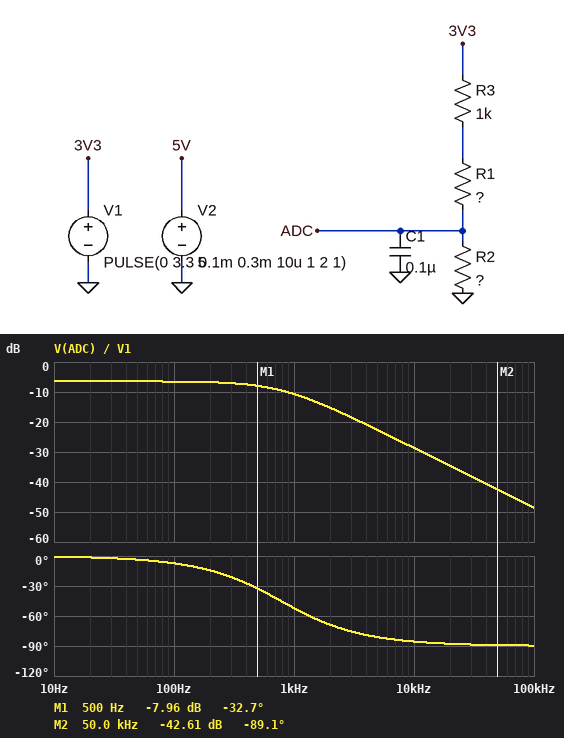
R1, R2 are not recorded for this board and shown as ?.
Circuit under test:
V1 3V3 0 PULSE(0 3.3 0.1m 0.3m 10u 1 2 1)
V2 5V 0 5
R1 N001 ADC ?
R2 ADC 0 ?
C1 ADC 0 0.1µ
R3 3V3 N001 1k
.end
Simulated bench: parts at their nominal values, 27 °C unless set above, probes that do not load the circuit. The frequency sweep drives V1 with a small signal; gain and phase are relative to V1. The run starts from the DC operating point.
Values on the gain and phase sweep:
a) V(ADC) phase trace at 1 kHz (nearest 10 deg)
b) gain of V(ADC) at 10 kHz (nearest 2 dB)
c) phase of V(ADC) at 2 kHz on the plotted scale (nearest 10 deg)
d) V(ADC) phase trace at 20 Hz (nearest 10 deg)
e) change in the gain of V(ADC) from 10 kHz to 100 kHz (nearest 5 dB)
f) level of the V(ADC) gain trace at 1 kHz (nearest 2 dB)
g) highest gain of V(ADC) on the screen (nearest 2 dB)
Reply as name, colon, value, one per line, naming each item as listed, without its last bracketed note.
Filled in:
V(ADC) phase trace at 1 kHz: -50 deg
gain of V(ADC) at 10 kHz: -28 dB
phase of V(ADC) at 2 kHz on the plotted scale: -70 deg
V(ADC) phase trace at 20 Hz: 0 deg
change in the gain of V(ADC) from 10 kHz to 100 kHz: -20 dB
level of the V(ADC) gain trace at 1 kHz: -10 dB
highest gain of V(ADC) on the screen: -6 dB
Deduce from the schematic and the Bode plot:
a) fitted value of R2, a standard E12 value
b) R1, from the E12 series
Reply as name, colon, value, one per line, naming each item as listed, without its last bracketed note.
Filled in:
fitted value of R2, a standard E12 value: 3.9 kΩ
R1, from the E12 series: 3.3 kΩ
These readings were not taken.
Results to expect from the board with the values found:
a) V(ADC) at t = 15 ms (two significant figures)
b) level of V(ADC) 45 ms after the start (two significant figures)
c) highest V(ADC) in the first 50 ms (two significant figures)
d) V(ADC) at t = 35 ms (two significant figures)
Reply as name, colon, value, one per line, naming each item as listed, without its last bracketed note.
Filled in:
V(ADC) at t = 15 ms: 1.6 V
level of V(ADC) 45 ms after the start: 1.6 V
highest V(ADC) in the first 50 ms: 1.6 V
V(ADC) at t = 35 ms: 1.6 V
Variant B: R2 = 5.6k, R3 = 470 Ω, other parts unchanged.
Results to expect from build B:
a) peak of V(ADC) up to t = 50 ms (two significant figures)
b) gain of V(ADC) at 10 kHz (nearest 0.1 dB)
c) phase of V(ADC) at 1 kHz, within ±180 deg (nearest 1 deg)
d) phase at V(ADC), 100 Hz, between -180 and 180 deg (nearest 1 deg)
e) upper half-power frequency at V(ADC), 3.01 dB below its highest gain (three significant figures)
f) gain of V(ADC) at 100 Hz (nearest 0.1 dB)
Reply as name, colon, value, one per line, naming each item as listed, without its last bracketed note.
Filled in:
peak of V(ADC) up to t = 50 ms: 2.0 V
gain of V(ADC) at 10 kHz: -27.5 dB
phase of V(ADC) at 1 kHz, within ±180 deg: -55 deg
phase at V(ADC), 100 Hz, between -180 and 180 deg: -8 deg
upper half-power frequency at V(ADC), 3.01 dB below its highest gain: 706 Hz
gain of V(ADC) at 100 Hz: -4.6 dB
